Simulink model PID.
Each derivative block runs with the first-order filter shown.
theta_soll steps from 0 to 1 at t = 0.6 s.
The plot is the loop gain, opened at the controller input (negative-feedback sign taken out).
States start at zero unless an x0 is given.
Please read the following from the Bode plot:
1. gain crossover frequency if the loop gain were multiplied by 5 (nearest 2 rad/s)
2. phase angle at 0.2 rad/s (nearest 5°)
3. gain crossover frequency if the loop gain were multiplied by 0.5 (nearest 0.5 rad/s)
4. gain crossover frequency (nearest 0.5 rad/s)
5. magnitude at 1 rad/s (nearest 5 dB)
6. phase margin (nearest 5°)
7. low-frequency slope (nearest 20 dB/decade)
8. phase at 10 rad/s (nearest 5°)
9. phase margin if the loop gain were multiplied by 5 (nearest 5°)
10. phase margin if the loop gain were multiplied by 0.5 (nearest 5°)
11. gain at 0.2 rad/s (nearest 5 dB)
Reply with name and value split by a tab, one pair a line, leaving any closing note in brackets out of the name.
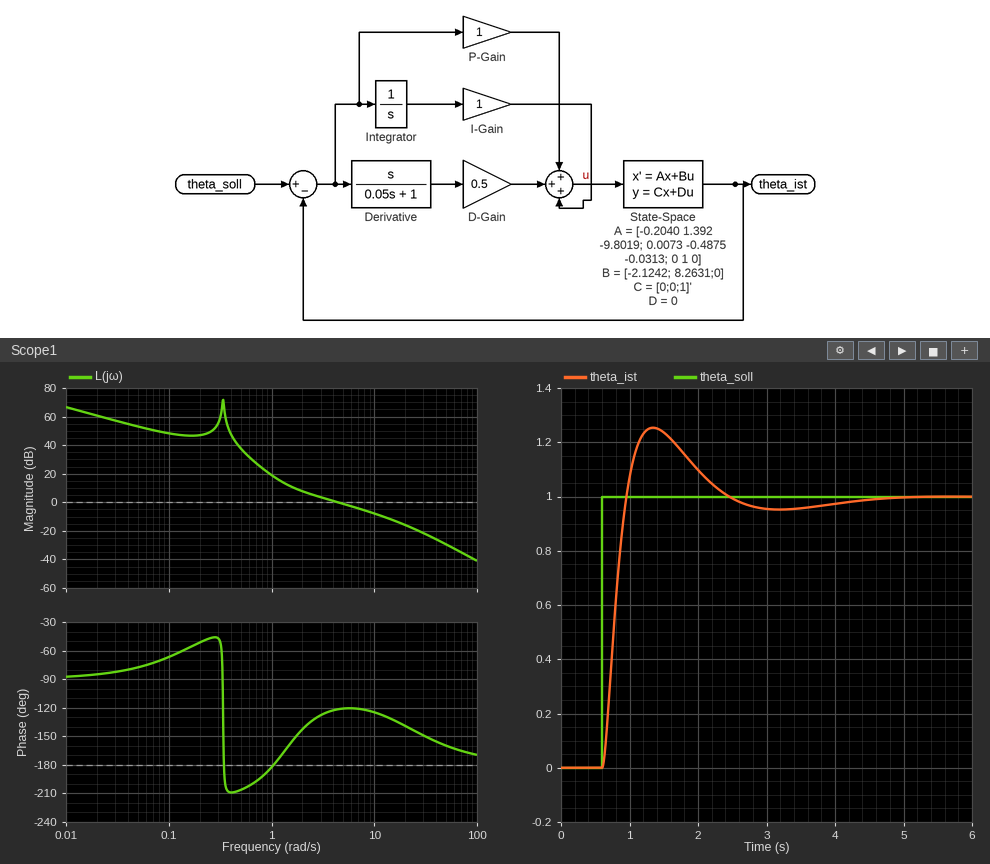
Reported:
gain crossover frequency if the loop gain were multiplied by 5	18 rad/s
phase angle at 0.2 rad/s	-50°
gain crossover frequency if the loop gain were multiplied by 0.5	2.5 rad/s
gain crossover frequency	4.5 rad/s
magnitude at 1 rad/s	20 dB
phase margin	60°
low-frequency slope	-20 dB/decade
phase at 10 rad/s	-125°
phase margin if the loop gain were multiplied by 5	45°
phase margin if the loop gain were multiplied by 0.5	45°
gain at 0.2 rad/s	45 dB
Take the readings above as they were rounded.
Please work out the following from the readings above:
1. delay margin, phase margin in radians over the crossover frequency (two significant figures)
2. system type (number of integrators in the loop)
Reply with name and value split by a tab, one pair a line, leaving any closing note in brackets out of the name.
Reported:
delay margin, phase margin in radians over the crossover frequency	0.23 s
system type	1
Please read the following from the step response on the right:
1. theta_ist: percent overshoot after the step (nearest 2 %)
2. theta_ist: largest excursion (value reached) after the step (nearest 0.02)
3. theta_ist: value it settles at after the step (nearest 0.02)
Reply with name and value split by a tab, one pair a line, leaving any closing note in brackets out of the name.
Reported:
theta_ist: percent overshoot after the step	26 %
theta_ist: largest excursion (value reached) after the step	1.26
theta_ist: value it settles at after the step	1.00
